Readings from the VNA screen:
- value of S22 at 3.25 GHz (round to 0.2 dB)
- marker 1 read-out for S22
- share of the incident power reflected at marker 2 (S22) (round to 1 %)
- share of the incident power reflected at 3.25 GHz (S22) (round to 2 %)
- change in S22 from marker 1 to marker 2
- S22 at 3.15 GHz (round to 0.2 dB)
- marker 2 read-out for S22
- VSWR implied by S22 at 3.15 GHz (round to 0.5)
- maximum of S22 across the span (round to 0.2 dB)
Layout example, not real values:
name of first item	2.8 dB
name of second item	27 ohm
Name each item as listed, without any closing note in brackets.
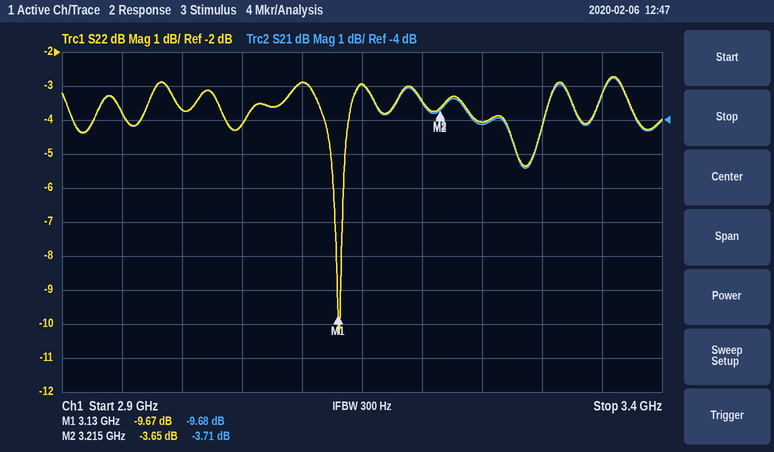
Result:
value of S22 at 3.25 GHz	-4.0 dB
marker 1 read-out for S22	-9.67 dB
share of the incident power reflected at marker 2 (S22)	43 %
share of the incident power reflected at 3.25 GHz (S22)	40 %
change in S22 from marker 1 to marker 2	6.02 dB
S22 at 3.15 GHz	-3.0 dB
marker 2 read-out for S22	-3.65 dB
VSWR implied by S22 at 3.15 GHz	6.0
maximum of S22 across the span	-2.8 dB
